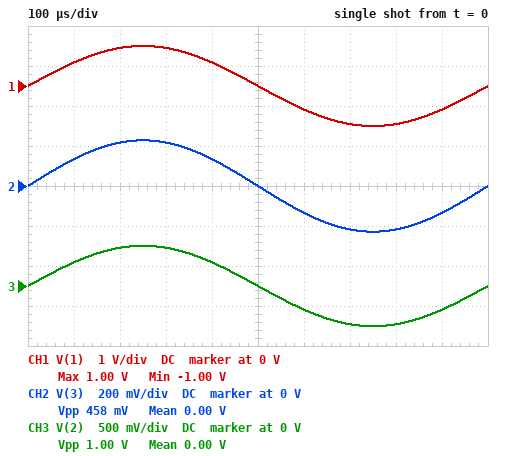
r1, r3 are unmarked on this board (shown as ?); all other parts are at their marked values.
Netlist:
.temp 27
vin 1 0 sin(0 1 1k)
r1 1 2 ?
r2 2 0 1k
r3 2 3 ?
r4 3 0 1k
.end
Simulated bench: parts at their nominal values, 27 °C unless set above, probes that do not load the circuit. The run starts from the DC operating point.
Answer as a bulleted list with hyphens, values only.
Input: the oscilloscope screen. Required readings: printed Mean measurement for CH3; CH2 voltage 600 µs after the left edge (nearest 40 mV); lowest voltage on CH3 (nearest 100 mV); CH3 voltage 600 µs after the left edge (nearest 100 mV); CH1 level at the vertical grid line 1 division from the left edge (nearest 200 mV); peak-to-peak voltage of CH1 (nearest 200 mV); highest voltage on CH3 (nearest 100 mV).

- 0.00 V
- -120 mV
- -500 mV
- -300 mV
- 600 mV
- 2.0 V
- 500 mV
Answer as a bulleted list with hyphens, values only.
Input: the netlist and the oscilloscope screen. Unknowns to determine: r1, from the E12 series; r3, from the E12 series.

- 680 Ω
- 1.2 kΩ
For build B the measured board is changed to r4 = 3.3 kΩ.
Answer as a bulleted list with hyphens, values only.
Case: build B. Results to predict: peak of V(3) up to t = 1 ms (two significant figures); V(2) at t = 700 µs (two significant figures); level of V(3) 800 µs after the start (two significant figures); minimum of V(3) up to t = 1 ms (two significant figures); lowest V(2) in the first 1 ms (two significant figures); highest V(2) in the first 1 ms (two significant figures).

- 400 mV
- -520 mV
- -380 mV
- -400 mV
- -550 mV
- 550 mV
